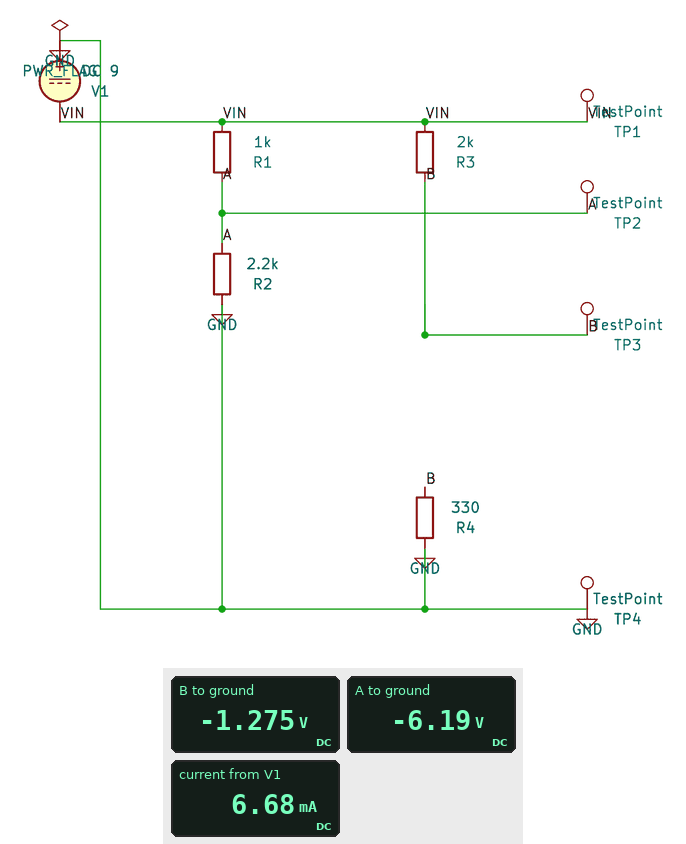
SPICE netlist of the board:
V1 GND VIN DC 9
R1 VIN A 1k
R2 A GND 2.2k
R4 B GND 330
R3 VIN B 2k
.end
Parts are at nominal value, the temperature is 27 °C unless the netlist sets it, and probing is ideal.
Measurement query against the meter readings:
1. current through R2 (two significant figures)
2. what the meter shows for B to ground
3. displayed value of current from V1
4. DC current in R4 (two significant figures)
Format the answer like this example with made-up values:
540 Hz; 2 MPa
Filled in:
2.8 mA; -1.275 V; 6.68 mA; 3.9 mA
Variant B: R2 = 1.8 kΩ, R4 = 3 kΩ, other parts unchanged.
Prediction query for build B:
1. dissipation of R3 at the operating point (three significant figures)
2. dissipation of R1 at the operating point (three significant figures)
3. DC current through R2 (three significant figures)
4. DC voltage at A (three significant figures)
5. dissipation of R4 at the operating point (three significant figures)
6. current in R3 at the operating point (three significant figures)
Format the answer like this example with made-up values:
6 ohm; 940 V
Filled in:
6.48 mW; 10.3 mW; 3.21 mA; -5.79 V; 9.72 mW; 1.80 mA
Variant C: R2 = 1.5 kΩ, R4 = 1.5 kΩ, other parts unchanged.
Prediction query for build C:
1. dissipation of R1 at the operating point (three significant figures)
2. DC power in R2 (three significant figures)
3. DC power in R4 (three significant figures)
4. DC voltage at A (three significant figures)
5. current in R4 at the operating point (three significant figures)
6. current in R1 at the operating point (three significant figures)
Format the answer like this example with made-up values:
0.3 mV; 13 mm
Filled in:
13.0 mW; 19.4 mW; 9.92 mW; -5.40 V; 2.57 mA; 3.60 mA
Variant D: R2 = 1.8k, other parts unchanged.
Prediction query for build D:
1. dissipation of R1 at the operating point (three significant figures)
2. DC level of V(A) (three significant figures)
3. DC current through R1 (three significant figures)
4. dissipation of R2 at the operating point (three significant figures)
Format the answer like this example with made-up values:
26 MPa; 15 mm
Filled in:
10.3 mW; -5.79 V; 3.21 mA; 18.6 mW
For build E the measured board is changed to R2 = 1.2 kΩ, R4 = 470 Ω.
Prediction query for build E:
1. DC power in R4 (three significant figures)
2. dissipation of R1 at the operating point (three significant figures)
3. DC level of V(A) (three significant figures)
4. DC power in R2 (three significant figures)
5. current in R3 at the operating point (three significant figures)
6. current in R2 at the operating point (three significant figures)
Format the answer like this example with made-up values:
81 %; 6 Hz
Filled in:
6.24 mW; 16.7 mW; -4.91 V; 20.1 mW; 3.64 mA; 4.09 mA
